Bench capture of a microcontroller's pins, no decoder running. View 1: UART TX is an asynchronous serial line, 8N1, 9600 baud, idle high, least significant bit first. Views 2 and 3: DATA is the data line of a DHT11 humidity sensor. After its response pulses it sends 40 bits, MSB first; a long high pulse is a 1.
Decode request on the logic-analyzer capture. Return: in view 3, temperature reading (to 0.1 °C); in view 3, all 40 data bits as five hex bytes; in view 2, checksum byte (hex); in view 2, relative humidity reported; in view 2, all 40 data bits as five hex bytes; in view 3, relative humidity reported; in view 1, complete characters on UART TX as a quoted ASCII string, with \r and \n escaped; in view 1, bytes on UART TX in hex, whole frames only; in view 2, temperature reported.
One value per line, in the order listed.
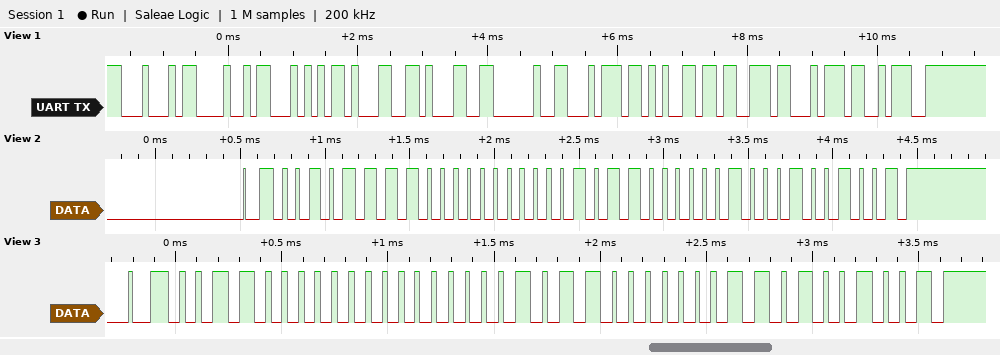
22.3 °C
30 00 16 03 49
0x49
47 %
2F 00 16 04 49
48 %
"DHT11 test:"
44 48 54 31 31 20 74 65 73 74 3A
22.4 °C
